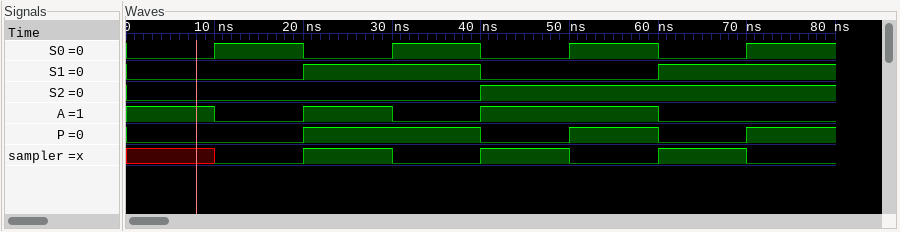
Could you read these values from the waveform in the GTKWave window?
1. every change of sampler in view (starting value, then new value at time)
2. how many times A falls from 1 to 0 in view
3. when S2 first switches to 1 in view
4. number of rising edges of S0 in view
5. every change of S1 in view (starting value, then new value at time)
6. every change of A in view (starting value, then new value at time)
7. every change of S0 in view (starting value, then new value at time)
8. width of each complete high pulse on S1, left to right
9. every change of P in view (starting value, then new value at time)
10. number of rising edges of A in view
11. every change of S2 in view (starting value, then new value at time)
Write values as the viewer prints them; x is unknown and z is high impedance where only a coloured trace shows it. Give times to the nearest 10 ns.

x, 0 at 10 ns, 1 at 20 ns, 0 at 30 ns, 1 at 40 ns, 0 at 50 ns, 1 at 60 ns, 0 at 70 ns
3
40 ns
4
0, 1 at 20 ns, 0 at 40 ns, 1 at 60 ns
1, 0 at 10 ns, 1 at 20 ns, 0 at 30 ns, 1 at 40 ns, 0 at 60 ns
0, 1 at 10 ns, 0 at 20 ns, 1 at 30 ns, 0 at 40 ns, 1 at 50 ns, 0 at 60 ns, 1 at 70 ns
20 ns
0, 1 at 20 ns, 0 at 40 ns, 1 at 50 ns, 0 at 60 ns, 1 at 70 ns
2
0, 1 at 40 ns
